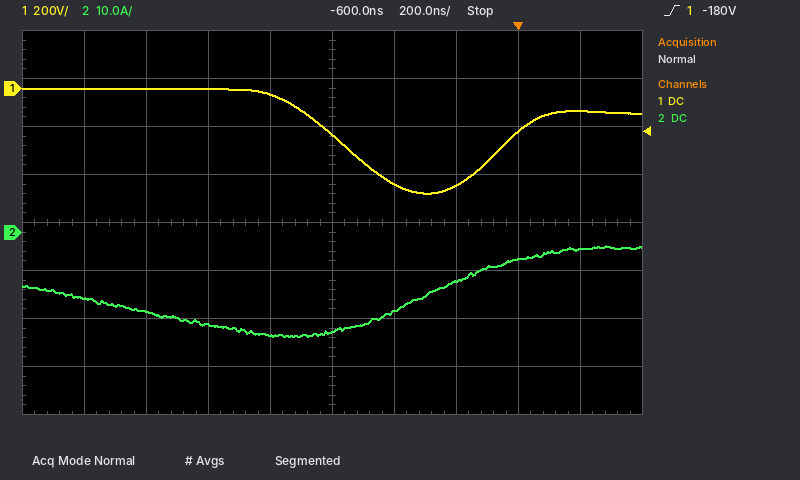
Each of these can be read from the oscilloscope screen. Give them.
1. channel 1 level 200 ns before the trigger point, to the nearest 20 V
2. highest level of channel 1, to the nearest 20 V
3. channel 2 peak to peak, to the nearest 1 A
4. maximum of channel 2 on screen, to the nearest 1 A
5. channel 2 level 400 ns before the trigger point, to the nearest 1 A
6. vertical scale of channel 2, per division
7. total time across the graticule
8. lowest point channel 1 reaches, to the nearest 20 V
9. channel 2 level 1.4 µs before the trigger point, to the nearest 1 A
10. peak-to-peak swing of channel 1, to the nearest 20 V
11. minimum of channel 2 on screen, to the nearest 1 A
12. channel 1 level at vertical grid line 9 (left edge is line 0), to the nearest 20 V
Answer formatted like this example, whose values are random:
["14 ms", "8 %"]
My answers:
["-400 V", "0 V", "19 A", "-3 A", "-17 A", "10 A", "2 µs", "-440 V", "-14 A", "440 V", "-22 A", "-100 V"]
